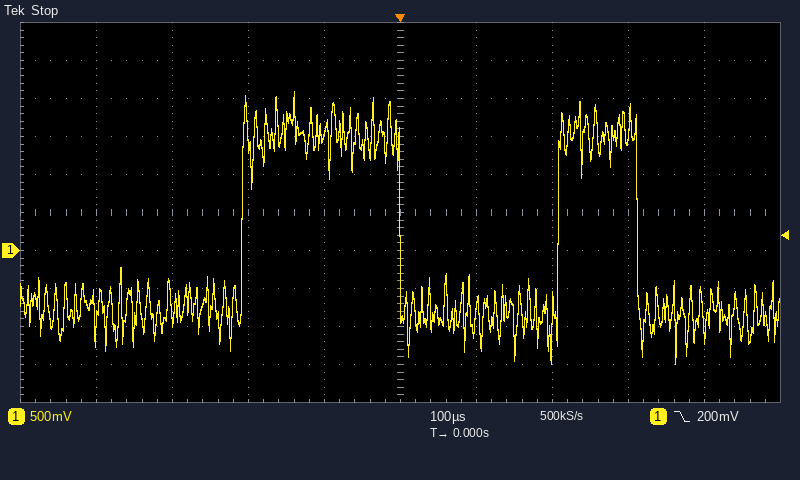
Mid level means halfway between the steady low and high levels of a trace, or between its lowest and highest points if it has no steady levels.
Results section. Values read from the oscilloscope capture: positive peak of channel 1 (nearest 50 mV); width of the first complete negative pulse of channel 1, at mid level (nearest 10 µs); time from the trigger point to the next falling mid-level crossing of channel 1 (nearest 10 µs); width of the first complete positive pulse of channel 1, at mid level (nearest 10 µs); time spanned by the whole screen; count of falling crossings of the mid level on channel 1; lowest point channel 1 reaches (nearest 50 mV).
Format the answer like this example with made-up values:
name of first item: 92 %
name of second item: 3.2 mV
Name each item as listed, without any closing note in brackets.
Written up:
positive peak of channel 1: 2.10 V
width of the first complete negative pulse of channel 1, at mid level: 210 µs
time from the trigger point to the next falling mid-level crossing of channel 1: 310 µs
width of the first complete positive pulse of channel 1, at mid level: 210 µs
time spanned by the whole screen: 1 ms
count of falling crossings of the mid level on channel 1: 2
lowest point channel 1 reaches: -1.50 V
